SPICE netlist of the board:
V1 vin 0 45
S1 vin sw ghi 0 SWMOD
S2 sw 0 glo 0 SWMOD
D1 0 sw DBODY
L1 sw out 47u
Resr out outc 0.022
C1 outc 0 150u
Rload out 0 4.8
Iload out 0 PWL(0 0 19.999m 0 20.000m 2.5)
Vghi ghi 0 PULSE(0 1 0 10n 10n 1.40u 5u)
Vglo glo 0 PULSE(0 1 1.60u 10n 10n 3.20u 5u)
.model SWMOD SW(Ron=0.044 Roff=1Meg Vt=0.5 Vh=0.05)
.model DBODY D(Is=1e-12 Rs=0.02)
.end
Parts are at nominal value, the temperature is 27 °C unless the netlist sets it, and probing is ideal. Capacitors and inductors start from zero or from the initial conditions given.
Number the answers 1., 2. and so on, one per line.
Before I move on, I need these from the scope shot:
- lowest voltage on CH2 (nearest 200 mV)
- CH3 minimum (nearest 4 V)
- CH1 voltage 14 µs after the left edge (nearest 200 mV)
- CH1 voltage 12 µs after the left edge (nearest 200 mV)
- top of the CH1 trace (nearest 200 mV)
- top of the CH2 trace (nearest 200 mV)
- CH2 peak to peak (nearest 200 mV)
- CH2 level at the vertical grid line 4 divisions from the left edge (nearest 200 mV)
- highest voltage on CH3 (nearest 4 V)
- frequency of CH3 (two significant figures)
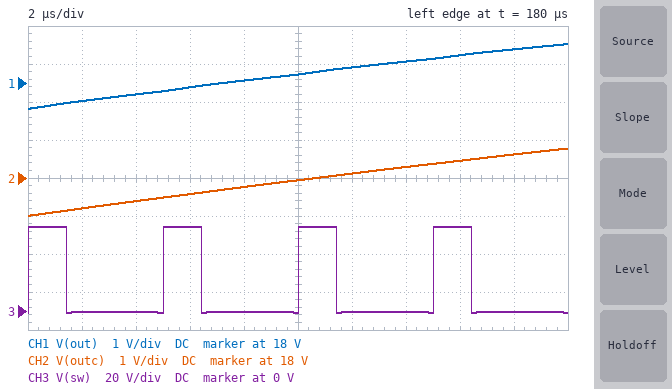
1. 17.0 V
2. 0 V
3. 18.6 V
4. 18.4 V
5. 19.0 V
6. 18.8 V
7. 1.8 V
8. 17.8 V
9. 44 V
10. 200 kHz
